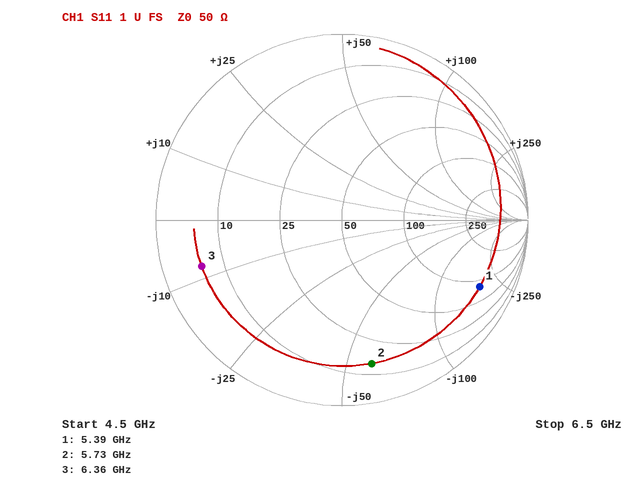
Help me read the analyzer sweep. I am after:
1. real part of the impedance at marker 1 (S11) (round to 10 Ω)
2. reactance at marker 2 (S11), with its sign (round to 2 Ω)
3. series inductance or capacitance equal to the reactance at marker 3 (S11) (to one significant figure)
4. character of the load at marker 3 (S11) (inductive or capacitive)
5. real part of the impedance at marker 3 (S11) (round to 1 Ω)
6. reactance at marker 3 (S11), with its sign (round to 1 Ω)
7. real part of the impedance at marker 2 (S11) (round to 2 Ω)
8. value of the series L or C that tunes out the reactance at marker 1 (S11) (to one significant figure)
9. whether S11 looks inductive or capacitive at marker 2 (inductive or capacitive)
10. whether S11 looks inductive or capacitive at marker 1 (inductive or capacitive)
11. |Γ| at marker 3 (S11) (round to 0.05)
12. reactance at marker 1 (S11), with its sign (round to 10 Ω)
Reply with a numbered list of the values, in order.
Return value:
1. 80 Ω
2. -60 Ω
3. 3 pF
4. capacitive
5. 6 Ω
6. -8 Ω
7. 14 Ω
8. 5 nH
9. capacitive
10. capacitive
11. 0.80
12. -180 Ω
